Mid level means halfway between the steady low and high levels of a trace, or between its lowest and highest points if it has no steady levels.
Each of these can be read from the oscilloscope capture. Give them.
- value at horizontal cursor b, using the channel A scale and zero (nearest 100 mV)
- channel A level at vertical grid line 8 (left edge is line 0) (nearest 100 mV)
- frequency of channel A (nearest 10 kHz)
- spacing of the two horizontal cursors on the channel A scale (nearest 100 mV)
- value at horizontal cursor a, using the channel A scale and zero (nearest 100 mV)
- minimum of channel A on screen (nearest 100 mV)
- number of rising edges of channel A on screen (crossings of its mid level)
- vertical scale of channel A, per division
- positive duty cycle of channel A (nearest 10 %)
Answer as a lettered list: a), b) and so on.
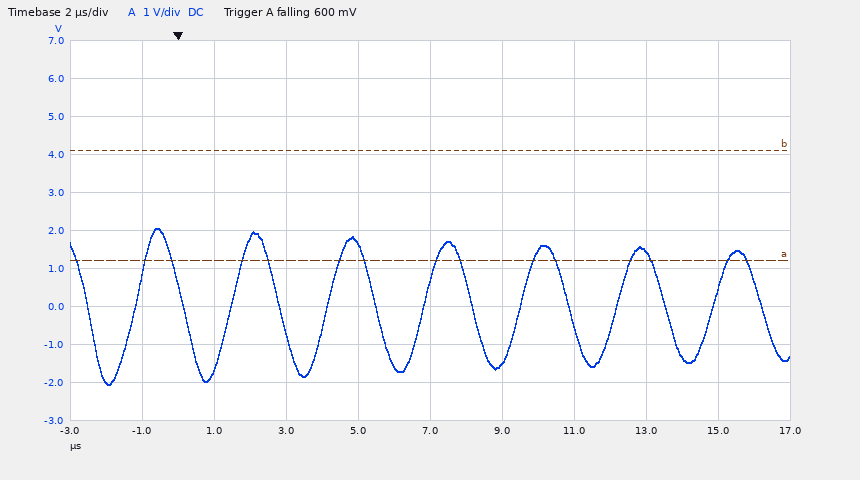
a) 4.1 V
b) 1.4 V
c) 370 kHz
d) 2.9 V
e) 1.2 V
f) -2.1 V
g) 7
h) 1 V
i) 50 %
